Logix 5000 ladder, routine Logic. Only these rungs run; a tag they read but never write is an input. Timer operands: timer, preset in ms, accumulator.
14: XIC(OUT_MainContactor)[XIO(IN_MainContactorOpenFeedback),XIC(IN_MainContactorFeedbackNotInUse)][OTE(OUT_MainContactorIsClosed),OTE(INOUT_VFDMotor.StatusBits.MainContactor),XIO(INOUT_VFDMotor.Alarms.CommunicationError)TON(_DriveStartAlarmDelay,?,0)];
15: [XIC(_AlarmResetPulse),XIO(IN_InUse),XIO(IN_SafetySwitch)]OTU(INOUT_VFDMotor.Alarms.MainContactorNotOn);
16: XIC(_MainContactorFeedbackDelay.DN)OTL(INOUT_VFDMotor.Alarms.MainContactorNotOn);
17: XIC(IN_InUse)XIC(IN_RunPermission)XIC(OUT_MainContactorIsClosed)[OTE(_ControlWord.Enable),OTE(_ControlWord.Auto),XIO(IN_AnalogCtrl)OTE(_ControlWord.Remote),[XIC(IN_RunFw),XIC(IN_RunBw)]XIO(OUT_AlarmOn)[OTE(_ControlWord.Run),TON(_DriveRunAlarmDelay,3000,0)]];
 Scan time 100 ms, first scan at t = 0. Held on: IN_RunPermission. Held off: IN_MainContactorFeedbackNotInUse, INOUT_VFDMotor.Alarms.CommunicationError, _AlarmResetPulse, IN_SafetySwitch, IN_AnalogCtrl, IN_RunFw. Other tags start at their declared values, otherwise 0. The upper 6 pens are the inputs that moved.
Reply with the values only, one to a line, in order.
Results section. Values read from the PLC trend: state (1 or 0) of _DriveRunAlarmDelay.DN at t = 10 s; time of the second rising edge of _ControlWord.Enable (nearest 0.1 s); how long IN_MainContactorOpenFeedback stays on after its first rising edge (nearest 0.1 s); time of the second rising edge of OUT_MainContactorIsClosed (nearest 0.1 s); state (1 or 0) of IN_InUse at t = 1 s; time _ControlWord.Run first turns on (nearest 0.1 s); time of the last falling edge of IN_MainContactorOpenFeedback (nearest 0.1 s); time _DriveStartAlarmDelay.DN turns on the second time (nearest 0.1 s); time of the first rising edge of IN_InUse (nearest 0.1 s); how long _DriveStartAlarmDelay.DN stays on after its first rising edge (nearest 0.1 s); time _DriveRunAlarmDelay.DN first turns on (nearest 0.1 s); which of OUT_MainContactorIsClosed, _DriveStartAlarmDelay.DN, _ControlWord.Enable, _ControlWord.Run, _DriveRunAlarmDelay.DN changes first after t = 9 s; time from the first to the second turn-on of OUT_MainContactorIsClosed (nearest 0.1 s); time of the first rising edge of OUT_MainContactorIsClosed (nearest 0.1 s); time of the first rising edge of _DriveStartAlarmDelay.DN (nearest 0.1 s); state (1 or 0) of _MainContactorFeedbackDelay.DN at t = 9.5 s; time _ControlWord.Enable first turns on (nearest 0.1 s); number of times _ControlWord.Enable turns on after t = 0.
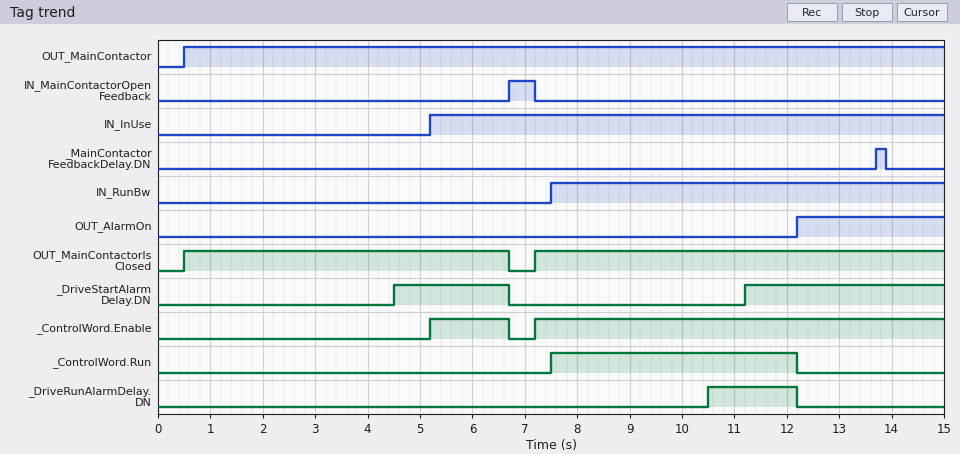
0
7.2 s
0.5 s
7.2 s
0
7.5 s
7.2 s
11.2 s
5.2 s
2.2 s
10.5 s
_DriveRunAlarmDelay.DN
6.7 s
0.5 s
4.5 s
0
5.2 s
2
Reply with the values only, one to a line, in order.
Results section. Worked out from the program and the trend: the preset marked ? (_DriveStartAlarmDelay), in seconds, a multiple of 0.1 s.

4.0 s
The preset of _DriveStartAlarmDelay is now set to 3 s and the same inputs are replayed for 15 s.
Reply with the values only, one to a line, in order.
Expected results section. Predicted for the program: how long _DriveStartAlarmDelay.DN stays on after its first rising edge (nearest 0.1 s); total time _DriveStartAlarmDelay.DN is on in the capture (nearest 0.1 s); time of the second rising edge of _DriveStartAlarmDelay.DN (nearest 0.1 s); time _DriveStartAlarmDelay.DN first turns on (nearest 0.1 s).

3.2 s
8.0 s
10.2 s
3.5 s
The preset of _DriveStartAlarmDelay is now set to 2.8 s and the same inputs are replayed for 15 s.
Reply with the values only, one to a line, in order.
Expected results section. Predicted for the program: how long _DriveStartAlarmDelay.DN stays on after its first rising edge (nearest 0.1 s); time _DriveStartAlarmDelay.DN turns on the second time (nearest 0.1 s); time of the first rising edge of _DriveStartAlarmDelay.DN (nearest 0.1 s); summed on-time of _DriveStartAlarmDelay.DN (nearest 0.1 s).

3.4 s
10.0 s
3.3 s
8.4 s
